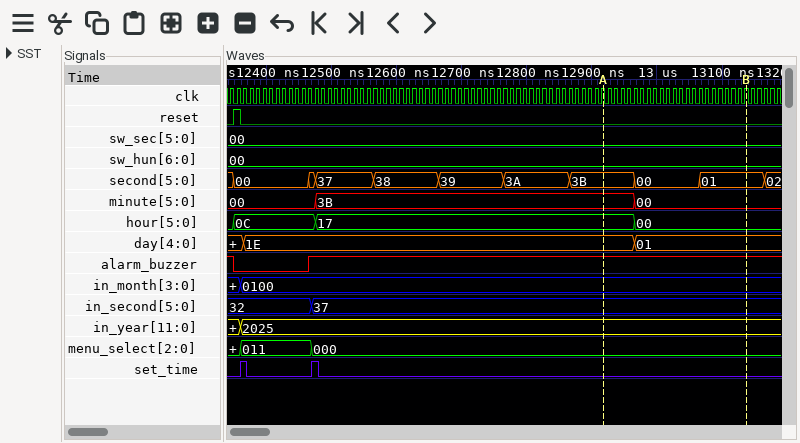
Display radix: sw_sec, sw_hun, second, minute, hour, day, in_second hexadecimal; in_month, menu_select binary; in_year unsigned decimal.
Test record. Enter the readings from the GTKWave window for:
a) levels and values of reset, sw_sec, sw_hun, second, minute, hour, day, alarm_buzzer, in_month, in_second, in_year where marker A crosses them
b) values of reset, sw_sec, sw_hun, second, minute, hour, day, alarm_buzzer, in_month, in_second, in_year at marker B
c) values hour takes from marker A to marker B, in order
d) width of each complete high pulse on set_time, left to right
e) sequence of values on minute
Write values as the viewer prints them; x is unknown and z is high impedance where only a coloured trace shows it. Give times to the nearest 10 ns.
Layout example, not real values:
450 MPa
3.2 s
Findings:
reset=0, sw_sec=00, sw_hun=00, second=3B, minute=3B, hour=17, day=1E, alarm_buzzer=1, in_month=0100, in_second=37, in_year=2025
reset=0, sw_sec=00, sw_hun=00, second=01, minute=00, hour=00, day=01, alarm_buzzer=1, in_month=0100, in_second=37, in_year=2025
17, 00
10 ns, 10 ns
00, 3B, 00
